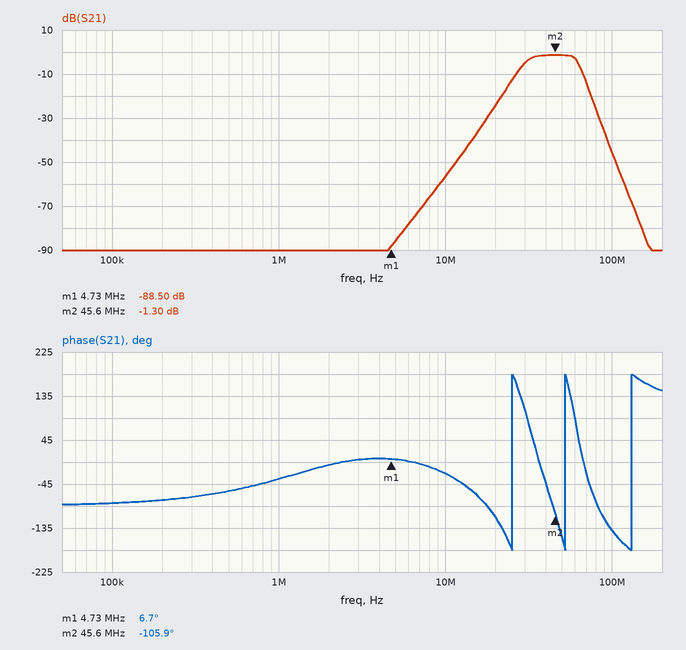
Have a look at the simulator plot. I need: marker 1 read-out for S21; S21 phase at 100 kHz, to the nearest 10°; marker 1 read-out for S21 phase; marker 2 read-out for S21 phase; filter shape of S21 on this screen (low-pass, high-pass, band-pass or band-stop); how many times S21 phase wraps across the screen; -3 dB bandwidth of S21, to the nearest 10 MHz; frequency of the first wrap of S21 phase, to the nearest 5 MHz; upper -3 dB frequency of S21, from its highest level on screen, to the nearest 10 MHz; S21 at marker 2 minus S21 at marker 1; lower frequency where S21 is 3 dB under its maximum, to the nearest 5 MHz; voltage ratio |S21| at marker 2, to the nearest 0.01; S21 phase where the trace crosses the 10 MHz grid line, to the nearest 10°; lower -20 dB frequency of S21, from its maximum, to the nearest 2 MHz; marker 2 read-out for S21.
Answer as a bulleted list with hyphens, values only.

- -88.50 dB
- -80°
- 6.7°
- -105.9°
- band-pass
- 3
- 30 MHz
- 25 MHz
- 60 MHz
- 87.20 dB
- 30 MHz
- 0.86
- -20°
- 22 MHz
- -1.30 dB
